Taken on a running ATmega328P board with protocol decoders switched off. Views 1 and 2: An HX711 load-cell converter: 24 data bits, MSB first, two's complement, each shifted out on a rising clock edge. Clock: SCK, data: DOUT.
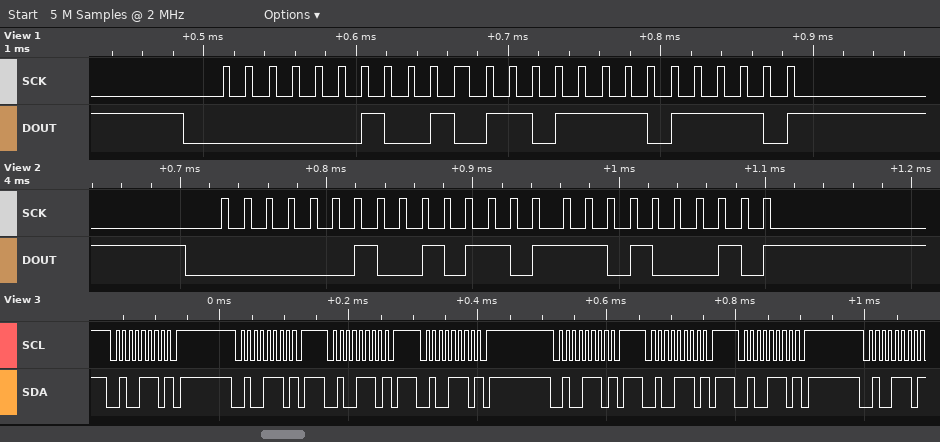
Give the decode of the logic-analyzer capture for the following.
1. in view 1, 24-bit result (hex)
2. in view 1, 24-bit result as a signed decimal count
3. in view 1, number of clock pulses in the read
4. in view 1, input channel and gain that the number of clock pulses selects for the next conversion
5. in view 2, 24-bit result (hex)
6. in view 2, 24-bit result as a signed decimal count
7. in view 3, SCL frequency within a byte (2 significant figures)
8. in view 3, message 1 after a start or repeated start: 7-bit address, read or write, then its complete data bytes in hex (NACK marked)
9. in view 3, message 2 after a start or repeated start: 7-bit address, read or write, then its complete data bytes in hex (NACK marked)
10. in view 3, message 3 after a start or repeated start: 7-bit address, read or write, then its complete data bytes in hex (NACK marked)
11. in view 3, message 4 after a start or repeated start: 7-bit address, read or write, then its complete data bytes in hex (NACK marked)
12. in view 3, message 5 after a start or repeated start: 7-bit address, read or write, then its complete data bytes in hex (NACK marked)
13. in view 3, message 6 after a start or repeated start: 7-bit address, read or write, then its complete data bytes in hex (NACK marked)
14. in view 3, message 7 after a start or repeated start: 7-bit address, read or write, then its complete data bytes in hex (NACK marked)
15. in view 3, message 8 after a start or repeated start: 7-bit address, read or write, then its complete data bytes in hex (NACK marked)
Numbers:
0x025BDE
154590
25
channel A, gain 128
0x025BA2
154530
100 kHz
0x27 write NACK
0x27 write NACK
0x27 write NACK
0x27 write NACK
0x27 write NACK
0x27 write NACK
0x27 write NACK
0x27 write NACK
